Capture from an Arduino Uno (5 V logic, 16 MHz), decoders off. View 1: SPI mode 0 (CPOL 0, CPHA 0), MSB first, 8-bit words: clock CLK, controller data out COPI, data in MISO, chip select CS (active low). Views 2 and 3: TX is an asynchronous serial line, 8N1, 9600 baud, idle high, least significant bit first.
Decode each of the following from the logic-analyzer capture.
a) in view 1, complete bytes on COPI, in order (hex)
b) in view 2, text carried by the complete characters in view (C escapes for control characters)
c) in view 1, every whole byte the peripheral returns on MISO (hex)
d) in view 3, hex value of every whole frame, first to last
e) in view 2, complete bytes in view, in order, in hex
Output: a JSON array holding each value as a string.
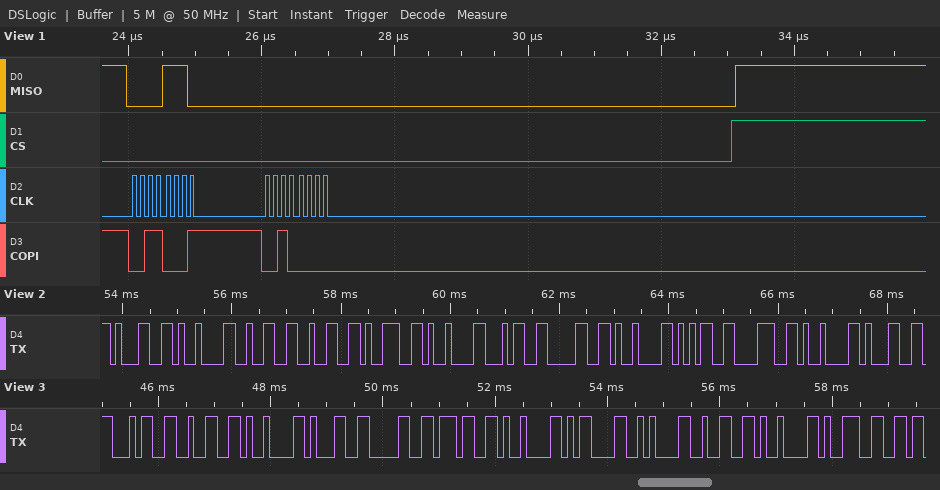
["31 20", "\"1\\t229\\t40\\t58\\t1\"", "0E 00", "0x34 0x32 0x09 0x31 0x30 0x37 0x09 0x0D 0x0A 0x32 0x09 0x39", "31 09 32 32 39 09 34 30 09 35 38 09 31"]
